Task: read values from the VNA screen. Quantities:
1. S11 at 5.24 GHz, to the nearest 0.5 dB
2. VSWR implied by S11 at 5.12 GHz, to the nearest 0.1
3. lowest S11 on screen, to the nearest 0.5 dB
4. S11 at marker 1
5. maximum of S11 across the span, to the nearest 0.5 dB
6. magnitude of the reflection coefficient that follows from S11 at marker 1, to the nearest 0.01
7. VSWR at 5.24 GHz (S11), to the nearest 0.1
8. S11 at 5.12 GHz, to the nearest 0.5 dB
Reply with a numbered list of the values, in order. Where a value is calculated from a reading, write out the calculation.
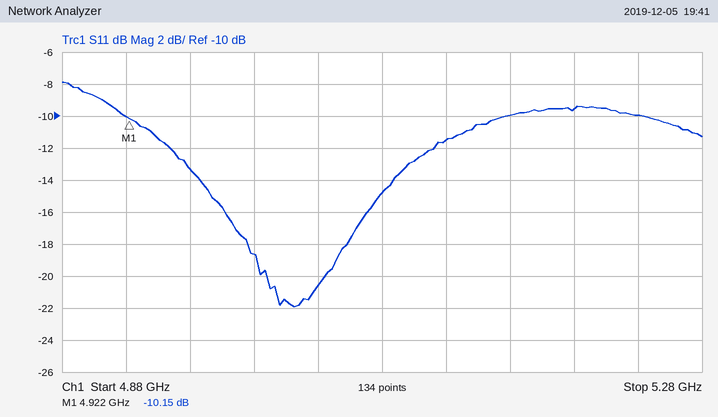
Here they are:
1. -10.0 dB
2. |Γ| = 10^(-11.5/20) = 0.2661; VSWR = (1 + 0.2661)/(1 − 0.2661) ≈ 1.7
3. -22.0 dB
4. -10.15 dB
5. -8.0 dB
6. 10^(-10.15/20) ≈ 0.31
7. |Γ| = 10^(-10/20) = 0.3162; VSWR = (1 + 0.3162)/(1 − 0.3162) ≈ 1.9
8. -11.5 dB
